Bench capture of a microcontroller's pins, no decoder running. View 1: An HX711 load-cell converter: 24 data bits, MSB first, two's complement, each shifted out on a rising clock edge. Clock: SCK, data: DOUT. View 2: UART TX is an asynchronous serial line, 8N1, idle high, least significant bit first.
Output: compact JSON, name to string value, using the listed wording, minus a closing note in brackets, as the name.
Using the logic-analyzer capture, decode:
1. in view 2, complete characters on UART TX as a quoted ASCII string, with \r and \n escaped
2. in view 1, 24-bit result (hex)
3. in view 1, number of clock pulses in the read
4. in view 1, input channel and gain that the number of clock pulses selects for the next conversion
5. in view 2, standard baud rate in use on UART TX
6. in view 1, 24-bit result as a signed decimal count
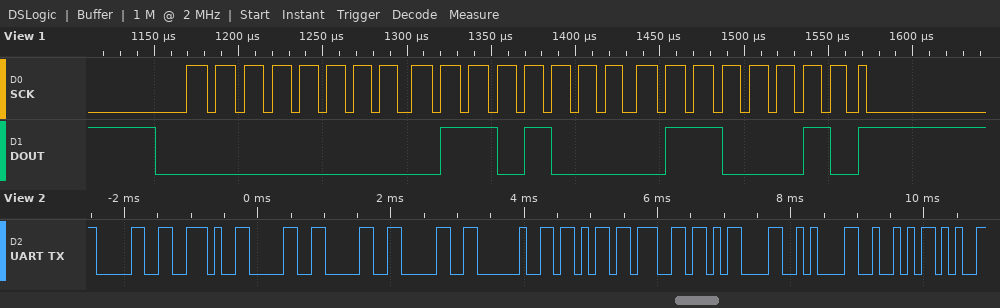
{"in view 2, complete characters on UART TX as a quoted ASCII string, with \\r and \\n escaped": "\"0.000 kg\\r\\nR\"", "in view 1, 24-bit result": "0x006862", "in view 1, number of clock pulses in the read": "25", "in view 1, input channel and gain that the number of clock pulses selects for the next conversion": "channel A, gain 128", "in view 2, standard baud rate in use on UART TX": "9600 baud", "in view 1, 24-bit result as a signed decimal count": "26722"}
